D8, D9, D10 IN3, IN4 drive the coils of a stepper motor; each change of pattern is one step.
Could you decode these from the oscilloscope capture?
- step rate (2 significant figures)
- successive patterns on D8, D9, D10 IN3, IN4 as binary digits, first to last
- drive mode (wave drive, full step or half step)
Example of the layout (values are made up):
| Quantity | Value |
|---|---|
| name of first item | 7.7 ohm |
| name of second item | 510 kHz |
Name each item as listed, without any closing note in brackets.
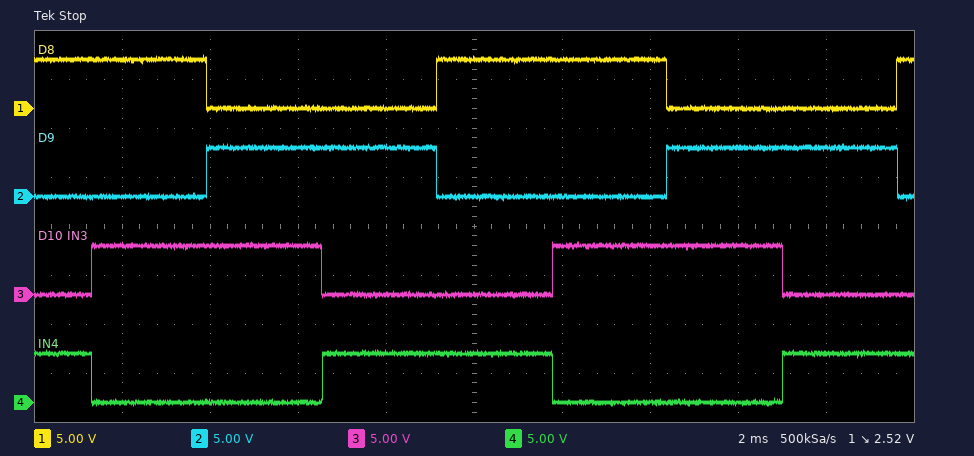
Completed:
| Quantity | Value |
|---|---|
| step rate | 380 steps/s |
| successive patterns on D8, D9, D10 IN3, IN4 as binary digits, first to last | 1001 1010 0110 0101 1001 1010 0110 0101 1001 |
| drive mode | full step |
